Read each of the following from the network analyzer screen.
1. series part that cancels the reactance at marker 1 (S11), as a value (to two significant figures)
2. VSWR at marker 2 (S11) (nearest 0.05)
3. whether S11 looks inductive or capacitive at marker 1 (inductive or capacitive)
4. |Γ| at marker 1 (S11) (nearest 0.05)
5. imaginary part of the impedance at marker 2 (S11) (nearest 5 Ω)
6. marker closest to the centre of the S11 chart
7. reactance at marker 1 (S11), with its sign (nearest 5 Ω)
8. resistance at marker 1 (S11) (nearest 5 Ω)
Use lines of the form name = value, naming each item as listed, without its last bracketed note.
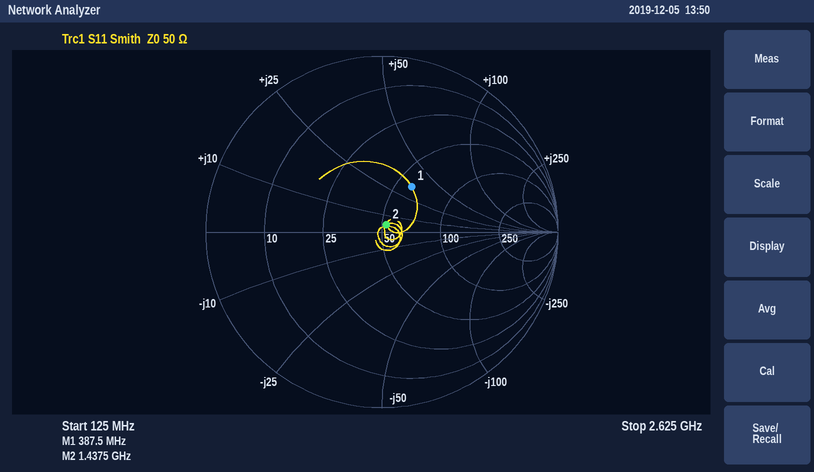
series part that cancels the reactance at marker 1 (S11), as a value = 12 pF
VSWR at marker 2 (S11) = 1.10
whether S11 looks inductive or capacitive at marker 1 = inductive
|Γ| at marker 1 (S11) = 0.30
imaginary part of the impedance at marker 2 (S11) = +5 Ω
marker closest to the centre of the S11 chart = marker 2
reactance at marker 1 (S11), with its sign = +35 Ω
resistance at marker 1 (S11) = 60 Ω
